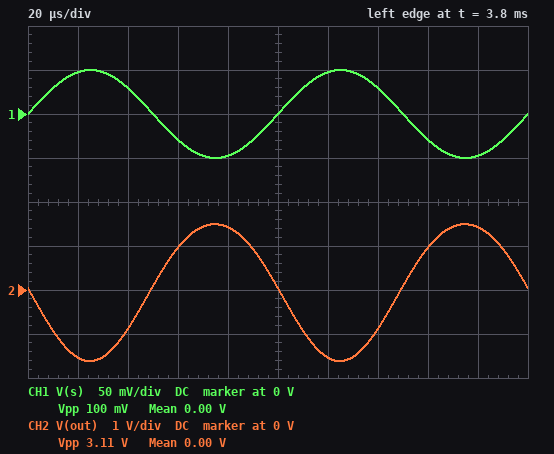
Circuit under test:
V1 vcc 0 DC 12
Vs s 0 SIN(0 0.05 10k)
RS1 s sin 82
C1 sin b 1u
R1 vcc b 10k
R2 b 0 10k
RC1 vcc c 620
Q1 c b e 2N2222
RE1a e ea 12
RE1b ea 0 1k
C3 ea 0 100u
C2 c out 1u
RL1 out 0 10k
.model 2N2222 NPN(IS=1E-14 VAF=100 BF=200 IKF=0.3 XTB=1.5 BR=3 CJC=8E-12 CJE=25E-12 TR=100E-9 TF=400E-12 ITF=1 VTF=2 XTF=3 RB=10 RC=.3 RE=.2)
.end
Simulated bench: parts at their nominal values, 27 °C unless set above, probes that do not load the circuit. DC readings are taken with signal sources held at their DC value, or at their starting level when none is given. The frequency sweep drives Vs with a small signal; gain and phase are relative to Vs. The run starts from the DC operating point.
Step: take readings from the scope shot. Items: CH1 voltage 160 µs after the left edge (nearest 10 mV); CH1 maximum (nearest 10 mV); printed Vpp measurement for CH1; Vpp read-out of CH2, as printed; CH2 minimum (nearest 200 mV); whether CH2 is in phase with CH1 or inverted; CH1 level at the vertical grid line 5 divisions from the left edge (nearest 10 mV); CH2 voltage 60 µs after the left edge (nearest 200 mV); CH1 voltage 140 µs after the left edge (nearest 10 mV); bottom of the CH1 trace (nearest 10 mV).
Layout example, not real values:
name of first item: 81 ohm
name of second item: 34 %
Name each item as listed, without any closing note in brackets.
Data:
CH1 voltage 160 µs after the left edge: -30 mV
CH1 maximum: 50 mV
printed Vpp measurement for CH1: 100 mV
Vpp read-out of CH2, as printed: 3.11 V
CH2 minimum: -1.6 V
whether CH2 is in phase with CH1 or inverted: inverted
CH1 level at the vertical grid line 5 divisions from the left edge: 0 V
CH2 voltage 60 µs after the left edge: 1.0 V
CH1 voltage 140 µs after the left edge: 30 mV
bottom of the CH1 trace: -50 mV
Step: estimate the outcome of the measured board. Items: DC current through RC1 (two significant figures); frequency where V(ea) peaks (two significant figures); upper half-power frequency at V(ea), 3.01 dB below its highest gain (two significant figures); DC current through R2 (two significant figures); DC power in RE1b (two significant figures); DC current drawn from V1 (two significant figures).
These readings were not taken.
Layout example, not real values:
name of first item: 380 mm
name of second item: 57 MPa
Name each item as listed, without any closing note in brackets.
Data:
DC current through RC1: 5.1 mA
frequency where V(ea) peaks: 54 Hz
upper half-power frequency at V(ea), 3.01 dB below its highest gain: 180 Hz
DC current through R2: 590 µA
DC power in RE1b: 26 mW
DC current drawn from V1: 5.7 mA
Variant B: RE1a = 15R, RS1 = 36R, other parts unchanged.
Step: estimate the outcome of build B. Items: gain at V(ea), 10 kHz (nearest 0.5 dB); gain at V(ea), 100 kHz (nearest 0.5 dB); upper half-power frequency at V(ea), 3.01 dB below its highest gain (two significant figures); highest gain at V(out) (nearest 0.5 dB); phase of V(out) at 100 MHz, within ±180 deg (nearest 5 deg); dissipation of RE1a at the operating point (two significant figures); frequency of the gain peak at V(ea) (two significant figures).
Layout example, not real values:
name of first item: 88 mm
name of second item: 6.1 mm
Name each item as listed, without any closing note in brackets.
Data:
gain at V(ea), 10 kHz: -42.5 dB
gain at V(ea), 100 kHz: -62.5 dB
upper half-power frequency at V(ea), 3.01 dB below its highest gain: 160 Hz
highest gain at V(out): 29.0 dB
phase of V(out) at 100 MHz, within ±180 deg: 80 deg
dissipation of RE1a at the operating point: 390 µW
frequency of the gain peak at V(ea): 50 Hz
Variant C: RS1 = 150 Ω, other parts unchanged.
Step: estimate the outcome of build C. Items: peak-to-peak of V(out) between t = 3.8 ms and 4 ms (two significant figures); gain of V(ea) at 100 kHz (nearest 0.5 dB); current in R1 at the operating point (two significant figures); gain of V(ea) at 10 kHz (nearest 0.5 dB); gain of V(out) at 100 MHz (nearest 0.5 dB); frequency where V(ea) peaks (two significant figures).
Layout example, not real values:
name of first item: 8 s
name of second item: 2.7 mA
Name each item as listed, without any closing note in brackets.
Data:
peak-to-peak of V(out) between t = 3.8 ms and 4 ms: 3.0 V
gain of V(ea) at 100 kHz: -61.5 dB
current in R1 at the operating point: 610 µA
gain of V(ea) at 10 kHz: -41.5 dB
gain of V(out) at 100 MHz: 3.5 dB
frequency where V(ea) peaks: 53 Hz
